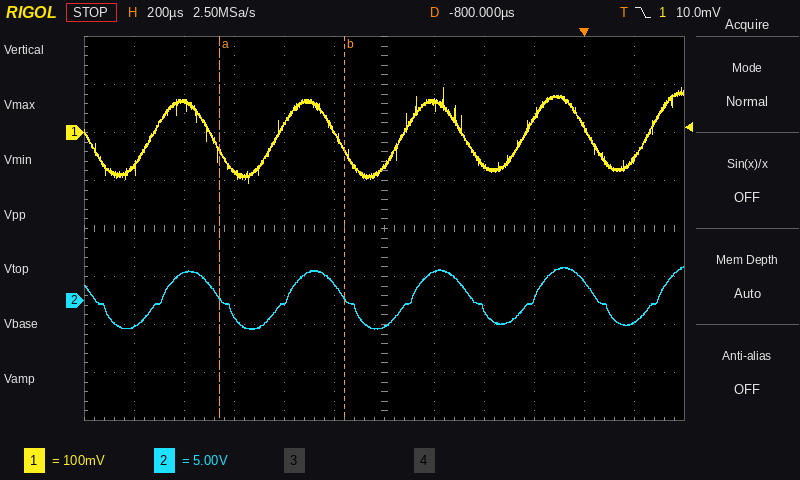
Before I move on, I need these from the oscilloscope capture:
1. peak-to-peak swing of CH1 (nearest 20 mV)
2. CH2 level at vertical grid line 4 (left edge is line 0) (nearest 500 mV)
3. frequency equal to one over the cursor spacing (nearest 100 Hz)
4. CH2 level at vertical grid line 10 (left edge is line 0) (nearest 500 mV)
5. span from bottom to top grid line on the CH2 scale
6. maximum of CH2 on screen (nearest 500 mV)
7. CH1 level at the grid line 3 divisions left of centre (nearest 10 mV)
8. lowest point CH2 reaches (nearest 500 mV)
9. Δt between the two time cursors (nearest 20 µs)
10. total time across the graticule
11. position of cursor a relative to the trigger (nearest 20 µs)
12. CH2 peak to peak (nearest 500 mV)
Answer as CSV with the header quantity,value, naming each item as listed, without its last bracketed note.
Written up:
quantity,value
peak-to-peak swing of CH1,200 mV
CH2 level at vertical grid line 4 (left edge is line 0),0.0 V
frequency equal to one over the cursor spacing,2.0 kHz
CH2 level at vertical grid line 10 (left edge is line 0),2.0 V
span from bottom to top grid line on the CH2 scale,40 V
maximum of CH2 on screen,3.5 V
CH1 level at the grid line 3 divisions left of centre,-80 mV
lowest point CH2 reaches,-3.0 V
Δt between the two time cursors,500 µs
total time across the graticule,2.4 ms
position of cursor a relative to the trigger,-1.46 ms
CH2 peak to peak,6.5 V
